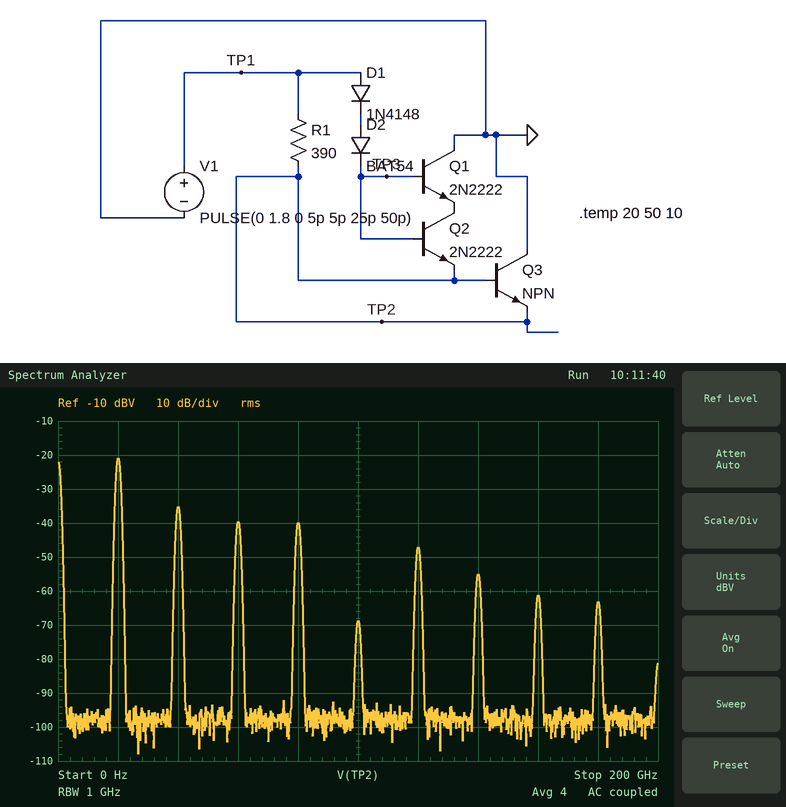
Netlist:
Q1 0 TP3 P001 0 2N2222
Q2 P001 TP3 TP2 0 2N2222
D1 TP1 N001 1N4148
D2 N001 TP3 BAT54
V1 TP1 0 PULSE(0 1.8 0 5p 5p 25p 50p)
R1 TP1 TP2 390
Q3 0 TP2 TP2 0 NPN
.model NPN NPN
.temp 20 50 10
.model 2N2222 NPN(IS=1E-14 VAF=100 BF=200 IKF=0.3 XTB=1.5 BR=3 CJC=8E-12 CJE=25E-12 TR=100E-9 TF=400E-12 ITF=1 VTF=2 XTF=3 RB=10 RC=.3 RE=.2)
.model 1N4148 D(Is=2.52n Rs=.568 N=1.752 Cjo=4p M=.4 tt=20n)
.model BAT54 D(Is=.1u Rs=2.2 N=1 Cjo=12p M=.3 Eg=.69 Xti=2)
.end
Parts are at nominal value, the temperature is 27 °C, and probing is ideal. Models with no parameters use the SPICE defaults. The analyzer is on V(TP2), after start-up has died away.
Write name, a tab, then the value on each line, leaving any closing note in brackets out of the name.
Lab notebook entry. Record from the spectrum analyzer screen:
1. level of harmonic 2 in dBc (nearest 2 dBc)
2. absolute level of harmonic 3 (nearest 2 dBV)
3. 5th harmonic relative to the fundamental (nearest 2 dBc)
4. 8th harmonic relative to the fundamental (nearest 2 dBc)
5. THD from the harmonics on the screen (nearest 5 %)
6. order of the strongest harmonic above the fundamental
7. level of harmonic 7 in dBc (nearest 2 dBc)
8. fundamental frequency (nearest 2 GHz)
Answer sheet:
level of harmonic 2 in dBc	-14 dBc
absolute level of harmonic 3	-40 dBV
5th harmonic relative to the fundamental	-48 dBc
8th harmonic relative to the fundamental	-40 dBc
THD from the harmonics on the screen	25 %
order of the strongest harmonic above the fundamental	2
level of harmonic 7 in dBc	-34 dBc
fundamental frequency	20 GHz
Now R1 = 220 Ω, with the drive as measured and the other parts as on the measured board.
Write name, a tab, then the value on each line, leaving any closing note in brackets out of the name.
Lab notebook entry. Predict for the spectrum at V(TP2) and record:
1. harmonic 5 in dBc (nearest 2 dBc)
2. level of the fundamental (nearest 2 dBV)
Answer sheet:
harmonic 5 in dBc	-46 dBc
level of the fundamental	-20 dBV
